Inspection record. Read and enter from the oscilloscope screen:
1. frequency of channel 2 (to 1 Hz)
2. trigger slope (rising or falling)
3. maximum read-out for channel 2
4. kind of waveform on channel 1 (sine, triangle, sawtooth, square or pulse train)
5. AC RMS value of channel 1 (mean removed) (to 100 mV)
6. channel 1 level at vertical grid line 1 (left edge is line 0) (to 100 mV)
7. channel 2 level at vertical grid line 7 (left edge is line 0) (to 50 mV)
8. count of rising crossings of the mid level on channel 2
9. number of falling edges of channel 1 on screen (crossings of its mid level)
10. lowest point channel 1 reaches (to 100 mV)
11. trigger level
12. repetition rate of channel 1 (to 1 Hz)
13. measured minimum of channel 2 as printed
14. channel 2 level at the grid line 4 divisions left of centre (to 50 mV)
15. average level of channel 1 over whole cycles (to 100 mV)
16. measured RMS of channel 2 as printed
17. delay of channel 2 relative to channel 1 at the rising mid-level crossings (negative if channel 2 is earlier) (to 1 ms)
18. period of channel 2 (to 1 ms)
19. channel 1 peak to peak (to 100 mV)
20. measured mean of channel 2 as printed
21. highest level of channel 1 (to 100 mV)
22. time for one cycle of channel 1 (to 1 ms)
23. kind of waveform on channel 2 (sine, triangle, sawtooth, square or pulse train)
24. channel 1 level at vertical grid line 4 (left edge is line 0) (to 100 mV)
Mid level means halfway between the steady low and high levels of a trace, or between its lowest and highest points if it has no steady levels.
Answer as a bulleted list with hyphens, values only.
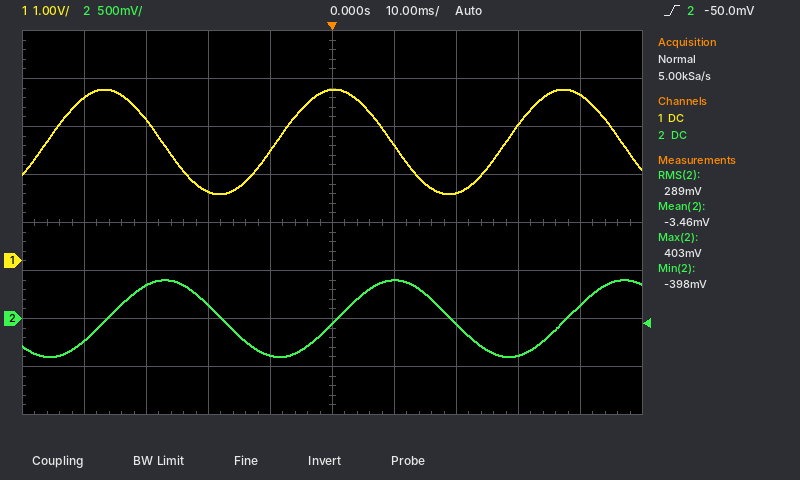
- 27 Hz
- rising
- 403 mV
- sine
- 800 mV
- 3.4 V
- -50 mV
- 3
- 3
- 1.4 V
- -50.0 mV
- 27 Hz
- -398 mV
- -250 mV
- 2.5 V
- 289 mV
- +10 ms
- 37 ms
- 2.2 V
- -3.46 mV
- 3.6 V
- 37 ms
- sine
- 2.3 V
